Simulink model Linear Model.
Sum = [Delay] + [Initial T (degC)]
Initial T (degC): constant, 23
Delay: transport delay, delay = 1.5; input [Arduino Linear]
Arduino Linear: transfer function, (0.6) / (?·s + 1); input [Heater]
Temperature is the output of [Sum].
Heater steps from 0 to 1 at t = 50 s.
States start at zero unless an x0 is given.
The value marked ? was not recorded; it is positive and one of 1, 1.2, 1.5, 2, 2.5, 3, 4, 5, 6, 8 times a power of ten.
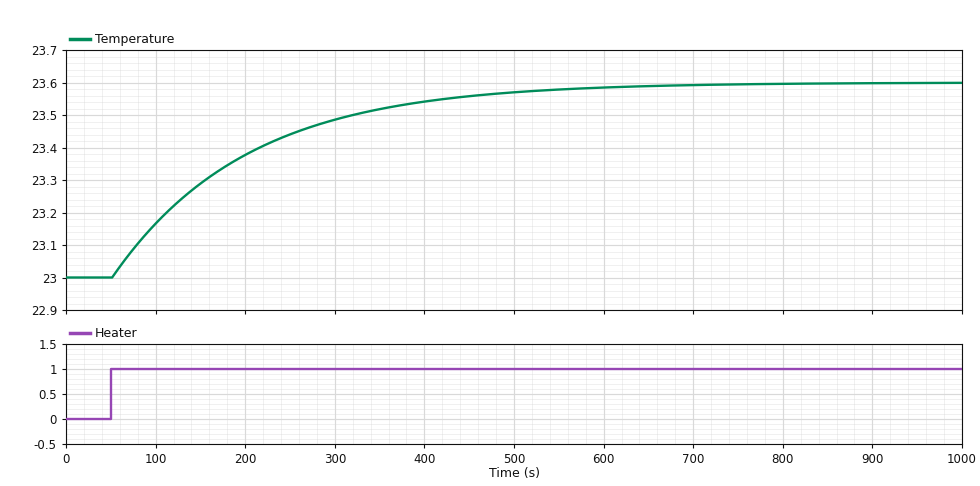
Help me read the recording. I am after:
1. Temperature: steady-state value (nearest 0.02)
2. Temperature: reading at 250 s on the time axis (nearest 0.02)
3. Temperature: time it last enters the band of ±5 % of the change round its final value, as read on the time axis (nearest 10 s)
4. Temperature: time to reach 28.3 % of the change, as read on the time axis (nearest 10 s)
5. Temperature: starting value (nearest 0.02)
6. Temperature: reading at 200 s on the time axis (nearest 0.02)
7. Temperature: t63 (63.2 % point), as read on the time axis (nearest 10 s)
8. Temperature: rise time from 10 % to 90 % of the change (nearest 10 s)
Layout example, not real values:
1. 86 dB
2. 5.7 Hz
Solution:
1. 23.60
2. 23.44
3. 500 s
4. 100 s
5. 23.00
6. 23.38
7. 200 s
8. 330 s
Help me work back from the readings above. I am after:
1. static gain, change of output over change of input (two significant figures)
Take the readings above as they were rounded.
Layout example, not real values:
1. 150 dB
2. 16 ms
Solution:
1. 0.60
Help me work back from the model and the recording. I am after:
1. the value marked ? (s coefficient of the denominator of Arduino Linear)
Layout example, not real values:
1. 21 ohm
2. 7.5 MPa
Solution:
1. 150
